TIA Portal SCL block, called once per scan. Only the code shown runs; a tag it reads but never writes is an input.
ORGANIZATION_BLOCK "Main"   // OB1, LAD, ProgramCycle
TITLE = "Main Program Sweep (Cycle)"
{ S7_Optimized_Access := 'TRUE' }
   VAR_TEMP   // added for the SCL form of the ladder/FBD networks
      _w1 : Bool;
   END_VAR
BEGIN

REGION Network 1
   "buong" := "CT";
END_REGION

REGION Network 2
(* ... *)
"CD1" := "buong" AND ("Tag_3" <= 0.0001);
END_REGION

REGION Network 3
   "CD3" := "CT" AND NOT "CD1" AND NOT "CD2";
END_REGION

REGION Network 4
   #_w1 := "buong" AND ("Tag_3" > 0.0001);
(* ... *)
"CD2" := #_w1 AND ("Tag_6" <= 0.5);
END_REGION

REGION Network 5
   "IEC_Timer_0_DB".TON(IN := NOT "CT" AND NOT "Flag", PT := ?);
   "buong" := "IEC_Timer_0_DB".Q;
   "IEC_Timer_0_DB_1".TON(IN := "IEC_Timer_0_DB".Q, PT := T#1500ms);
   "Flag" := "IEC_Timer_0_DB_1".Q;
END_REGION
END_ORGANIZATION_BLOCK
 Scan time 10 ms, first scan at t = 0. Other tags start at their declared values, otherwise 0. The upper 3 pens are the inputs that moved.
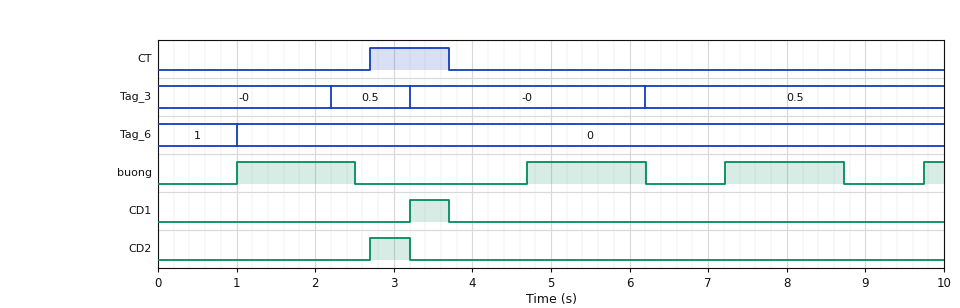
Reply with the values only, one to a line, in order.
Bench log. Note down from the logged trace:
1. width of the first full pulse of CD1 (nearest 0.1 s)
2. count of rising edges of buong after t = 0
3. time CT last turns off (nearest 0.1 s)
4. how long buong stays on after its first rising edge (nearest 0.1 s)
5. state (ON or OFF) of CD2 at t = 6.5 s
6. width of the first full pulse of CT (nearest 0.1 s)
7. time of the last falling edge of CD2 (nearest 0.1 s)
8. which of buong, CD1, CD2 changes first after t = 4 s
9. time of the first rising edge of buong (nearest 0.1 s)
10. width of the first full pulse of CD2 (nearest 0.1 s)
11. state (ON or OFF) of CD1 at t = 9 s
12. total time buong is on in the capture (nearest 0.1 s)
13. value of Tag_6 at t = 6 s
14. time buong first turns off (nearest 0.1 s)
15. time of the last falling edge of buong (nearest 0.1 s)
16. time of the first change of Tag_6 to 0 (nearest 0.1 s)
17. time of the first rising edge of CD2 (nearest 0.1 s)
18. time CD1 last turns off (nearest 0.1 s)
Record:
0.5 s
4
3.7 s
1.5 s
OFF
1.0 s
3.2 s
buong
1.0 s
0.5 s
OFF
4.8 s
0
2.5 s
8.7 s
1.0 s
2.7 s
3.7 s
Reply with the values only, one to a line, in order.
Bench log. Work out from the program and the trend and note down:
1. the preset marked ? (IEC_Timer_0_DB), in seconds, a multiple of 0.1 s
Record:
1.0 s
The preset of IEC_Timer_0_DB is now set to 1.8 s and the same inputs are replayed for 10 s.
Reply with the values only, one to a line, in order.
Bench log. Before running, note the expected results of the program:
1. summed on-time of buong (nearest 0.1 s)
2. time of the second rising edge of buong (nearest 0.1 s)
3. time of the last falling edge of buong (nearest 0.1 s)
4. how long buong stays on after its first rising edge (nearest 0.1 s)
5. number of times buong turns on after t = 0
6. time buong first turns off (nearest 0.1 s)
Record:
3.6 s
5.5 s
7.0 s
0.9 s
3
2.7 s
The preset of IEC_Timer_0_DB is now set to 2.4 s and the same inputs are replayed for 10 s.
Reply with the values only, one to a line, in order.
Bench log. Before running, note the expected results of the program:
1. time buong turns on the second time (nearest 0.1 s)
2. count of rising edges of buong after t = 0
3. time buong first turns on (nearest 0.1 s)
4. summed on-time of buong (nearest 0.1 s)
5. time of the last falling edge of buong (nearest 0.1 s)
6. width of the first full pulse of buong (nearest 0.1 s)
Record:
6.1 s
2
2.4 s
1.8 s
7.6 s
0.3 s
